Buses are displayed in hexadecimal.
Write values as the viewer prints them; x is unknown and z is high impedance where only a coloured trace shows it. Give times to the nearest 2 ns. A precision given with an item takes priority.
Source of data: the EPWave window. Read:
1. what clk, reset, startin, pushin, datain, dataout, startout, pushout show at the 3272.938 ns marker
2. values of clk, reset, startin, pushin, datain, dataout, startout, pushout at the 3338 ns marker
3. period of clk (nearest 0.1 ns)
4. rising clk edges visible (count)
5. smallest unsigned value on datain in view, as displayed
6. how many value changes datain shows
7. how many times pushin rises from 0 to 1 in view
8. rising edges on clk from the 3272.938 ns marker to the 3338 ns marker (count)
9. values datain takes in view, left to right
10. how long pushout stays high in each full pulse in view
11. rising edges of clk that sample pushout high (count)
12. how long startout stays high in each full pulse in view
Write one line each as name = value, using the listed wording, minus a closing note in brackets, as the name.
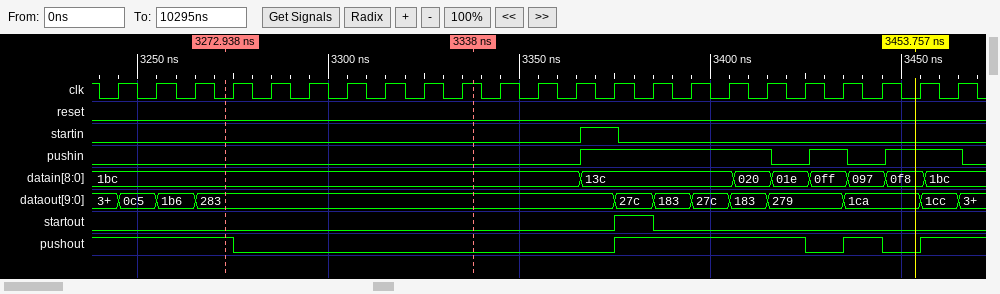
what clk, reset, startin, pushin, datain, dataout, startout, pushout show at the 3272.938 ns marker = clk=0, reset=0, startin=0, pushin=0, datain=1bc, dataout=283, startout=0, pushout=1
values of clk, reset, startin, pushin, datain, dataout, startout, pushout at the 3338 ns marker = clk=1, reset=0, startin=0, pushin=0, datain=1bc, dataout=283, startout=0, pushout=0
period of clk = 10 ns
rising clk edges visible = 23
smallest unsigned value on datain in view, as displayed = 01e
how many value changes datain shows = 7
how many times pushin rises from 0 to 1 in view = 3
rising edges on clk from the 3272.938 ns marker to the 3338 ns marker = 7
values datain takes in view, left to right = 1bc, 13c, 020, 01e, 0ff, 097, 0f8, 1bc
how long pushout stays high in each full pulse in view = 50 ns, 10 ns
rising edges of clk that sample pushout high = 11
how long startout stays high in each full pulse in view = 10 ns
